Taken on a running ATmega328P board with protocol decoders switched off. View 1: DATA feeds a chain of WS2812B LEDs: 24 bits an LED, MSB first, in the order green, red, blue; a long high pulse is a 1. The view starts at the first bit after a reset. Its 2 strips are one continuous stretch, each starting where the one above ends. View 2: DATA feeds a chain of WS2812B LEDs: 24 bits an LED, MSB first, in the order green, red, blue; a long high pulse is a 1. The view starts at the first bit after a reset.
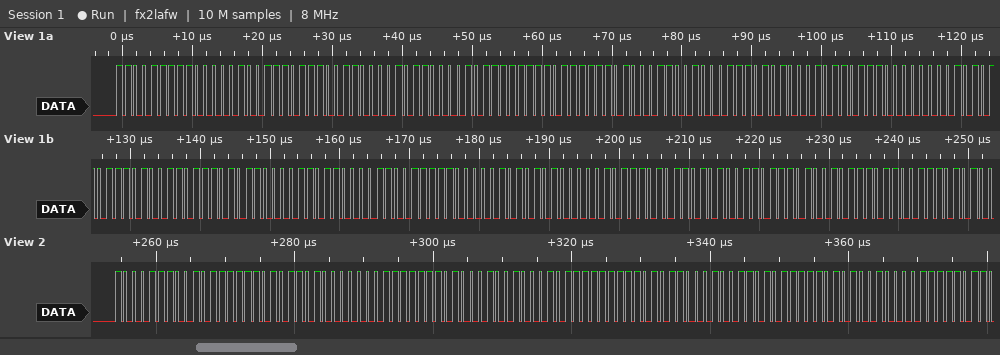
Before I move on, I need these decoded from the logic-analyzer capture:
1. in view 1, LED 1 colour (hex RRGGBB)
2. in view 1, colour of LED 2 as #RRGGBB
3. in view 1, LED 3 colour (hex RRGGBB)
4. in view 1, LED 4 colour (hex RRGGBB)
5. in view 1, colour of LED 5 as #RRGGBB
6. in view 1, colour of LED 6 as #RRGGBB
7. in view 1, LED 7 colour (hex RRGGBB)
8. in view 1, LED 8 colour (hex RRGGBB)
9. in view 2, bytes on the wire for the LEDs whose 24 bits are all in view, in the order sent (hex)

#82CF77
#B030BF
#A3DF23
#B7A800
#A6ABEB
#860D7C
#411575
#BAA95D
8E 5F AD 01 FD 12 2F FA C4 D7 D4 87
